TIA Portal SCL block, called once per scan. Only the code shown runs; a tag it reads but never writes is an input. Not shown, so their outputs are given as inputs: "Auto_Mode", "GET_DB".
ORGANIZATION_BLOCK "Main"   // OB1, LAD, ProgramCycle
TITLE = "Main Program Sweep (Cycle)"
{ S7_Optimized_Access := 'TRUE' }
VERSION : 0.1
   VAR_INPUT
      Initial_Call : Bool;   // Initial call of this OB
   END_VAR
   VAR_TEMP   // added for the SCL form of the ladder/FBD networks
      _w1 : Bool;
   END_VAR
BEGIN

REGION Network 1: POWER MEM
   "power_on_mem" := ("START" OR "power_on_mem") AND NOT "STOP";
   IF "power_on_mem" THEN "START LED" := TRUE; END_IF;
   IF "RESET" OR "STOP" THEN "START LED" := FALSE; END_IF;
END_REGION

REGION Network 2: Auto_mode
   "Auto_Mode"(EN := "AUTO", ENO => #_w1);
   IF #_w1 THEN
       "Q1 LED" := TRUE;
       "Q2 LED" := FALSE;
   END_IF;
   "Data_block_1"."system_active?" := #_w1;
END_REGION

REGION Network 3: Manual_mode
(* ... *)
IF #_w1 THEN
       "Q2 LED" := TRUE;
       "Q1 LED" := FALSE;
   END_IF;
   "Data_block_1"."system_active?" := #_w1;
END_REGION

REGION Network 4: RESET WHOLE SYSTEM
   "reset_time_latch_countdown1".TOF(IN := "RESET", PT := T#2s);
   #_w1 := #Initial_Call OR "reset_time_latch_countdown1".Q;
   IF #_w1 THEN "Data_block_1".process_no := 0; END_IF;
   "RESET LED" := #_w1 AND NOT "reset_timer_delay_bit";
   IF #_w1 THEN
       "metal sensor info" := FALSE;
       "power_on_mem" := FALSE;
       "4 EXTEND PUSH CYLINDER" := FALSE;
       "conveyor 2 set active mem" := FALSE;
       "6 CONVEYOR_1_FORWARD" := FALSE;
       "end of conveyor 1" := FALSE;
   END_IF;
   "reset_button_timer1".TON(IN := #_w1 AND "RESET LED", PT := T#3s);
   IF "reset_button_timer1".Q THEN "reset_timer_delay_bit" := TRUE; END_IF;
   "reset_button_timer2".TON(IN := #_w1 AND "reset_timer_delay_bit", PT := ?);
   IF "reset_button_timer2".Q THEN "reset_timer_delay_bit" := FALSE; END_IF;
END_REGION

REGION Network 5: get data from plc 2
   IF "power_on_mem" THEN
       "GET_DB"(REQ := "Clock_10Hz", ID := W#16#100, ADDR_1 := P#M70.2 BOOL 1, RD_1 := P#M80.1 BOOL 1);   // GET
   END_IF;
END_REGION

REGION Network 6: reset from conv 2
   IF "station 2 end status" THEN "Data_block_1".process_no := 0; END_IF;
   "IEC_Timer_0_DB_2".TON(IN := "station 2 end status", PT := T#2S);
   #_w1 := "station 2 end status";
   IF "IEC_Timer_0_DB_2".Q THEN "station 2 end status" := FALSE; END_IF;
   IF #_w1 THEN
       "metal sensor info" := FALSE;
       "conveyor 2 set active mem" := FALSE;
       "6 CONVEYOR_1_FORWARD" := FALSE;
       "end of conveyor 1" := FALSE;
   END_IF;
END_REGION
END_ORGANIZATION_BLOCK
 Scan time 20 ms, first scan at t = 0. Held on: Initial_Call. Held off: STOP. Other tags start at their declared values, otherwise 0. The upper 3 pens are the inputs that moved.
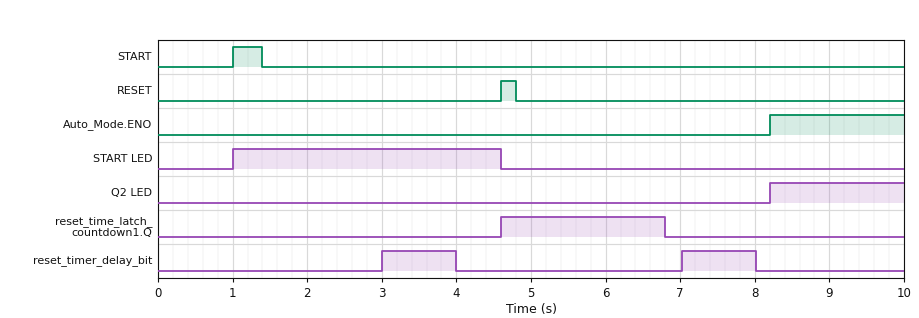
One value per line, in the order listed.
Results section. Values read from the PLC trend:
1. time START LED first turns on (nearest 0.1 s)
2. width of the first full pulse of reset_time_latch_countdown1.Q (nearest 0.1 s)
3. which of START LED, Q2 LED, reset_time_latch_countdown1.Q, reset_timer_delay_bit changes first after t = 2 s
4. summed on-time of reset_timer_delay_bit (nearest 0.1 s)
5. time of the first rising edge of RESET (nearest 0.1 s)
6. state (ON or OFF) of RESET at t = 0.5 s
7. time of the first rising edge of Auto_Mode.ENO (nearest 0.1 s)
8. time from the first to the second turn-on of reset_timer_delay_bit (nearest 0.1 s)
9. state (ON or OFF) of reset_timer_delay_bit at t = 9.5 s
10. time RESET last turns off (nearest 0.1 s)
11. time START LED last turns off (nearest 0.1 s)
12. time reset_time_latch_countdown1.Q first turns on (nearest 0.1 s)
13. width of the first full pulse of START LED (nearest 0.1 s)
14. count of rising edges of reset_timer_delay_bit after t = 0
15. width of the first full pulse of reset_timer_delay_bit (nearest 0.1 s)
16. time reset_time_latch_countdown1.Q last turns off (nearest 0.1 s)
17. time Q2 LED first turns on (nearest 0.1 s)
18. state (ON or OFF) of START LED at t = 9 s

1.0 s
2.2 s
reset_timer_delay_bit
2.0 s
4.6 s
OFF
8.2 s
4.0 s
OFF
4.8 s
4.6 s
4.6 s
3.6 s
2
1.0 s
6.8 s
8.2 s
OFF
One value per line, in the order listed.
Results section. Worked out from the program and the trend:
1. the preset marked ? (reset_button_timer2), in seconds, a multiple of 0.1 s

1.0 s
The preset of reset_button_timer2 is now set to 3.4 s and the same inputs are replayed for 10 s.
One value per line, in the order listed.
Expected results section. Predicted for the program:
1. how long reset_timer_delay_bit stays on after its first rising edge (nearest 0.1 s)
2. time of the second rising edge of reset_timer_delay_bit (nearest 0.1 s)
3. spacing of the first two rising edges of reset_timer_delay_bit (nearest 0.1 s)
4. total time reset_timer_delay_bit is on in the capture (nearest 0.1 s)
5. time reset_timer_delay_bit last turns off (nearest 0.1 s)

3.4 s
9.4 s
6.4 s
4.0 s
6.4 s
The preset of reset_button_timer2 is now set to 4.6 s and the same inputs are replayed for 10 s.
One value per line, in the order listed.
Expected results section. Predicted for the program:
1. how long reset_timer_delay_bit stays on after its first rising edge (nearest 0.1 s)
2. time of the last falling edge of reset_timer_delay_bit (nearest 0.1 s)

4.6 s
7.6 s
